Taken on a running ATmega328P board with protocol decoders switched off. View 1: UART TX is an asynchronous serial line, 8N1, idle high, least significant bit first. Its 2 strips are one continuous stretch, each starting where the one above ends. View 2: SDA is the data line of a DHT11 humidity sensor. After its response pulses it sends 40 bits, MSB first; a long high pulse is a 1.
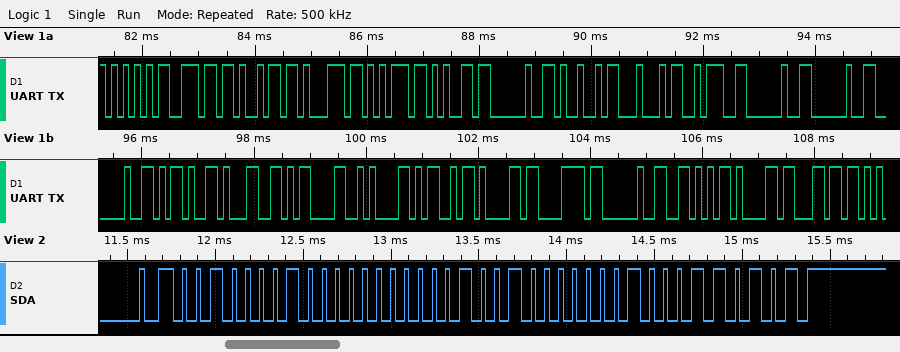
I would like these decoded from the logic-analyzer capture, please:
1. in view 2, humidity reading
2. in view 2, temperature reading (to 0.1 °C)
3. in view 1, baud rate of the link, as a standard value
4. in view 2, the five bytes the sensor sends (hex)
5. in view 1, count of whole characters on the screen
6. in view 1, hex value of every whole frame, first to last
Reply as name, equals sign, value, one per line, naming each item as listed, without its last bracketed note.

in view 2, humidity reading = 33 %
in view 2, temperature reading = 18.2 °C
in view 1, baud rate of the link, as a standard value = 9600 baud
in view 2, the five bytes the sensor sends = 21 00 12 02 35
in view 1, count of whole characters on the screen = 24
in view 1, hex value of every whole frame, first to last = 55 6E 69 71 75 65 20 49 44 3A 20 20 20 2D 31 0D 0A 4D 61 78 20 56 61 6C
